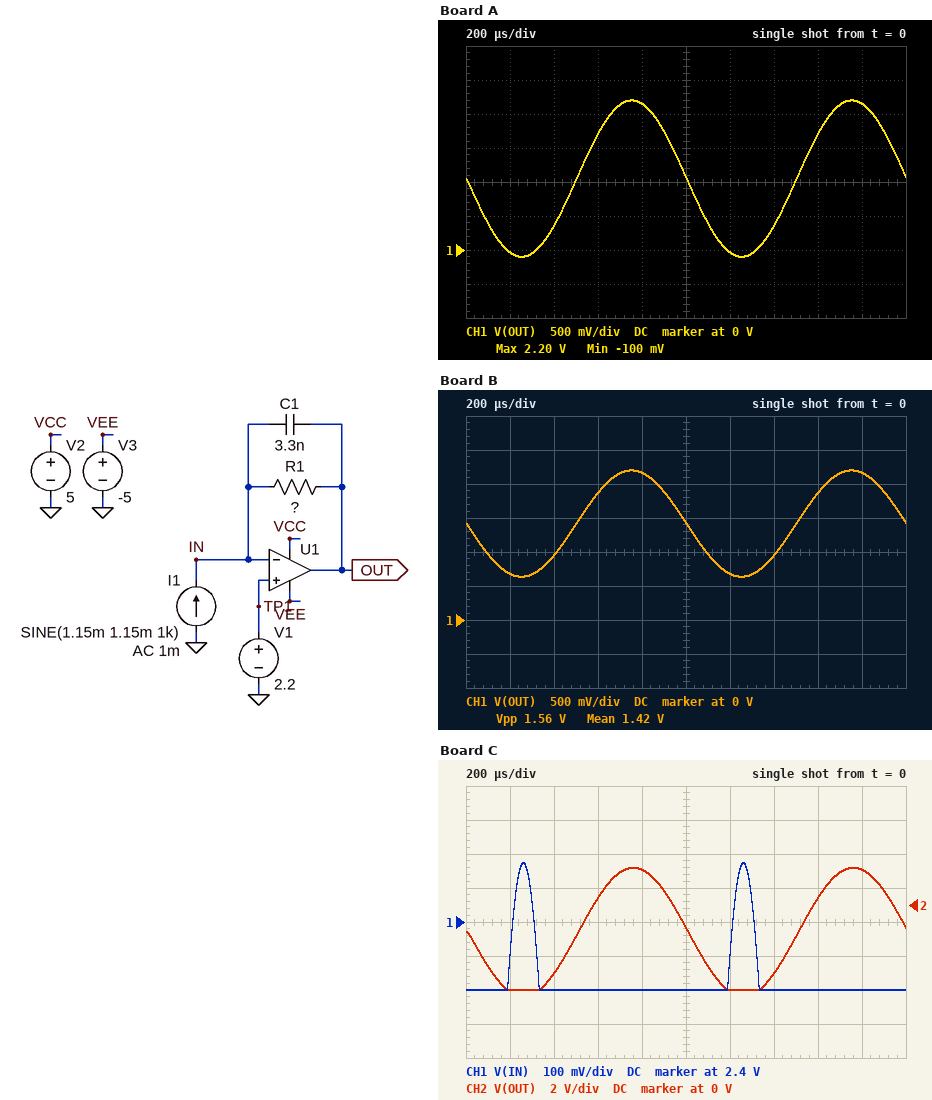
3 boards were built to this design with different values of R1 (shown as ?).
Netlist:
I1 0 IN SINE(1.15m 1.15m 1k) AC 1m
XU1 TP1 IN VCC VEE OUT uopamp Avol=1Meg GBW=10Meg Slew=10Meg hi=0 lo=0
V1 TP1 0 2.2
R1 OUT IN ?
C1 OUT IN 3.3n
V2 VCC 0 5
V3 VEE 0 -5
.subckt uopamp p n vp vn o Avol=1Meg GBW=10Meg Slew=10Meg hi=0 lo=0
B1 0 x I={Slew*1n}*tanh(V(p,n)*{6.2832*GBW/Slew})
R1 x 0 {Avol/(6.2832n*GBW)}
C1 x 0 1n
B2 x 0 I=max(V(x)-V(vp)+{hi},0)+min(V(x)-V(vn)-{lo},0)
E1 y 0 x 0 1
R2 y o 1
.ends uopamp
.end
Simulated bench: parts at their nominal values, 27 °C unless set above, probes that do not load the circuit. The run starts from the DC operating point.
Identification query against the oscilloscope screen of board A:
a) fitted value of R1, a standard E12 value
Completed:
1 kΩ
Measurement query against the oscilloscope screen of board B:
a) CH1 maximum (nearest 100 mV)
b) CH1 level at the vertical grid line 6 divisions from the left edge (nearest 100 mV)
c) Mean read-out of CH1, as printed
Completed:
2.2 V
700 mV
1.42 V
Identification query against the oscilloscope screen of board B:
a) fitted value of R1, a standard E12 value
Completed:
680 Ω
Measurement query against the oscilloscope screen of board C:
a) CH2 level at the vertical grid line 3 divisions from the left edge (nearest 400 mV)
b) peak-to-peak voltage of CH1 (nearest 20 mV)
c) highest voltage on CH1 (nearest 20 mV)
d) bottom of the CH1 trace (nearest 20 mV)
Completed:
400 mV
380 mV
2.58 V
2.20 V
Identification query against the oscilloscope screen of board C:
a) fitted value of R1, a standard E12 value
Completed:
3.3 kΩ
